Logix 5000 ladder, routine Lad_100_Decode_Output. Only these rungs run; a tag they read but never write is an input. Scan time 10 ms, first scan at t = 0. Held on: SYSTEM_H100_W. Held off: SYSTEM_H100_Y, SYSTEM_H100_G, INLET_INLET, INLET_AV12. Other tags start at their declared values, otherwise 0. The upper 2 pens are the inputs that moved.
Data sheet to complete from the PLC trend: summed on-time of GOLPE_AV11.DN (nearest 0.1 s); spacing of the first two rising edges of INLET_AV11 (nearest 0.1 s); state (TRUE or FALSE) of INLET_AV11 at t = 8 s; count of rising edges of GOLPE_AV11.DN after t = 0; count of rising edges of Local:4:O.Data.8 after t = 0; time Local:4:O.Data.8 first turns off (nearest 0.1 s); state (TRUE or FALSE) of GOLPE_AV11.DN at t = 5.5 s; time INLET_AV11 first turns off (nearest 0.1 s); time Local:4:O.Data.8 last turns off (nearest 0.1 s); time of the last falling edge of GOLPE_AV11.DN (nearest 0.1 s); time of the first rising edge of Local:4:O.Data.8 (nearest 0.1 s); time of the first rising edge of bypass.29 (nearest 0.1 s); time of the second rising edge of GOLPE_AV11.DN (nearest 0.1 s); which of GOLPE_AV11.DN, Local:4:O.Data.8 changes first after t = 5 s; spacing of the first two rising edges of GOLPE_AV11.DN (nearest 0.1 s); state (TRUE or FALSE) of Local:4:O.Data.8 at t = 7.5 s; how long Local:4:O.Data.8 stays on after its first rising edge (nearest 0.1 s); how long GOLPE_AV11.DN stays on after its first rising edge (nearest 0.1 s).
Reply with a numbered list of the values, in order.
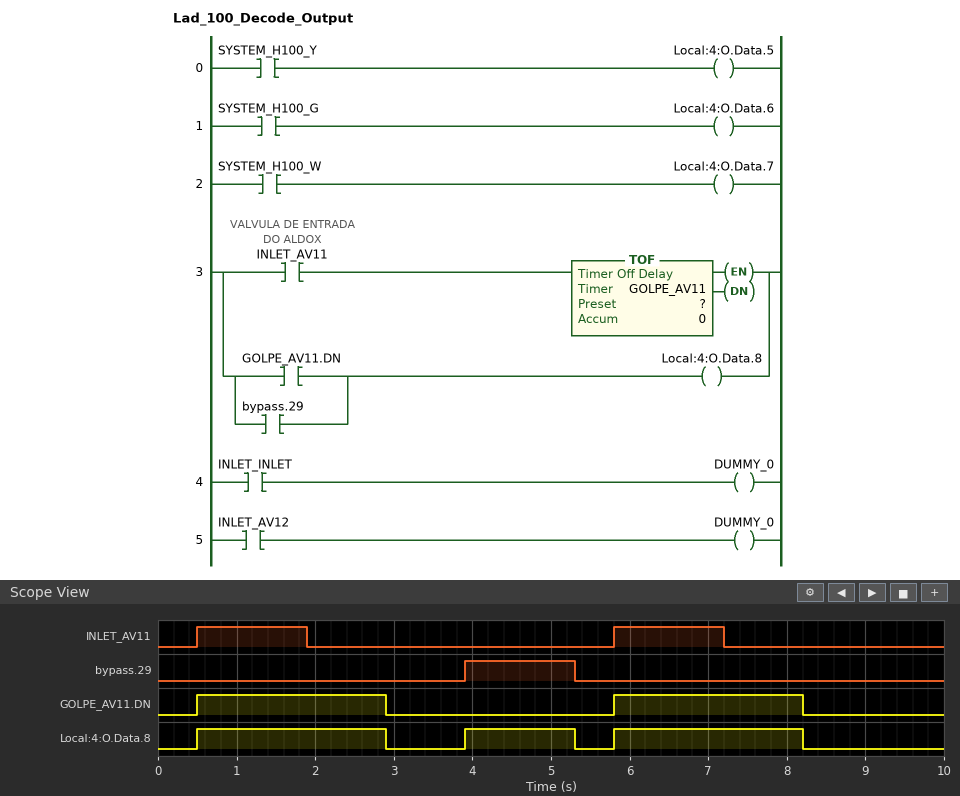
1. 4.8 s
2. 5.3 s
3. FALSE
4. 2
5. 3
6. 2.9 s
7. FALSE
8. 1.9 s
9. 8.2 s
10. 8.2 s
11. 0.5 s
12. 3.9 s
13. 5.8 s
14. Local:4:O.Data.8
15. 5.3 s
16. TRUE
17. 2.4 s
18. 2.4 s
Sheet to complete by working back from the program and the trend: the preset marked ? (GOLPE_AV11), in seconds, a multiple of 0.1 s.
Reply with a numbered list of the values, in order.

1. 1.0 s
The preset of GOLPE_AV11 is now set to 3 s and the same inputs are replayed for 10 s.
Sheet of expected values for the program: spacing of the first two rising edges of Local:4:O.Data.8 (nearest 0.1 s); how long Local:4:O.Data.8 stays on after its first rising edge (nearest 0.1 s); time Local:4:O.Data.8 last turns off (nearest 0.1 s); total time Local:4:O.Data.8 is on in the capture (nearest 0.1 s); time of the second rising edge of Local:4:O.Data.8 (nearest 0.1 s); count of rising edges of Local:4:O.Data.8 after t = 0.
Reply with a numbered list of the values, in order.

1. 5.3 s
2. 4.8 s
3. 5.3 s
4. 9.0 s
5. 5.8 s
6. 2
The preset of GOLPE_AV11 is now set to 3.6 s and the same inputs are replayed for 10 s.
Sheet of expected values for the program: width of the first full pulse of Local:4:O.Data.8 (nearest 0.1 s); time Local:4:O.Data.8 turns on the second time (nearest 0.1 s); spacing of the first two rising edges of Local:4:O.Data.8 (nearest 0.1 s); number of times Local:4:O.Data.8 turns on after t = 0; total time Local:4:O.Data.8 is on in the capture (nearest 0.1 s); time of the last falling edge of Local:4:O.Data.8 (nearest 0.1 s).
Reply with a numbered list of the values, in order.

1. 5.0 s
2. 5.8 s
3. 5.3 s
4. 2
5. 9.2 s
6. 5.5 s
